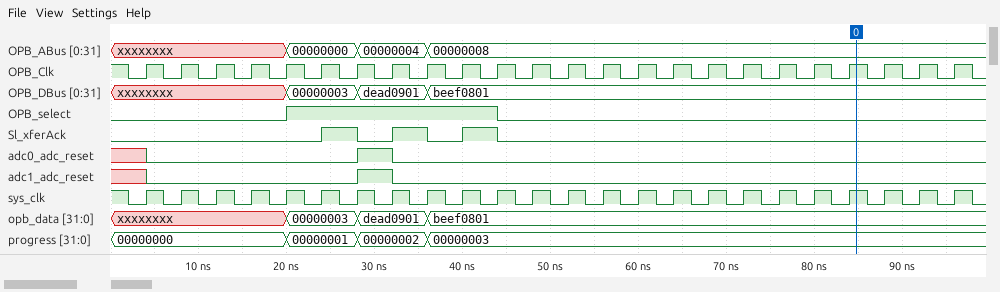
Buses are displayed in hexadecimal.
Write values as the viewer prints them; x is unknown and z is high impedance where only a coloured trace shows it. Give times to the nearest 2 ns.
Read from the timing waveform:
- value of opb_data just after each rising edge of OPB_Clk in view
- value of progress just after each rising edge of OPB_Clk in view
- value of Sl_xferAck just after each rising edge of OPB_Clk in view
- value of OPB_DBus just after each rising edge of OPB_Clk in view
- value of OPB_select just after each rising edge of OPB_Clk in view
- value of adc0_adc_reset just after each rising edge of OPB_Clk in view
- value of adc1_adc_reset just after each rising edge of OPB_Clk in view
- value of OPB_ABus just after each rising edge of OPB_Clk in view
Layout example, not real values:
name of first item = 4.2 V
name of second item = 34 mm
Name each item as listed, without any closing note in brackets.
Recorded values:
value of opb_data just after each rising edge of OPB_Clk in view = xxxxxxxx, xxxxxxxx, xxxxxxxx, xxxxxxxx, 00000003, 00000003, dead0901, dead0901, beef0801, beef0801, beef0801, beef0801, beef0801, beef0801, beef0801, beef0801, beef0801, beef0801, beef0801, beef0801, beef0801, beef0801, beef0801, beef0801
value of progress just after each rising edge of OPB_Clk in view = 00000000, 00000000, 00000000, 00000000, 00000001, 00000001, 00000002, 00000002, 00000003, 00000003, 00000003, 00000003, 00000003, 00000003, 00000003, 00000003, 00000003, 00000003, 00000003, 00000003, 00000003, 00000003, 00000003, 00000003
value of Sl_xferAck just after each rising edge of OPB_Clk in view = 0 0 0 0 0 1 0 1 0 1 0 0 0 0 0 0 0 0 0 0 0 0 0 0
value of OPB_DBus just after each rising edge of OPB_Clk in view = xxxxxxxx, xxxxxxxx, xxxxxxxx, xxxxxxxx, 00000003, 00000003, dead0901, dead0901, beef0801, beef0801, beef0801, beef0801, beef0801, beef0801, beef0801, beef0801, beef0801, beef0801, beef0801, beef0801, beef0801, beef0801, beef0801, beef0801
value of OPB_select just after each rising edge of OPB_Clk in view = 0 0 0 0 1 1 1 1 1 1 0 0 0 0 0 0 0 0 0 0 0 0 0 0
value of adc0_adc_reset just after each rising edge of OPB_Clk in view = 0 0 0 0 0 0 1 0 0 0 0 0 0 0 0 0 0 0 0 0 0 0 0 0
value of adc1_adc_reset just after each rising edge of OPB_Clk in view = 0 0 0 0 0 0 1 0 0 0 0 0 0 0 0 0 0 0 0 0 0 0 0 0
value of OPB_ABus just after each rising edge of OPB_Clk in view = xxxxxxxx, xxxxxxxx, xxxxxxxx, xxxxxxxx, 00000000, 00000000, 00000004, 00000004, 00000008, 00000008, 00000008, 00000008, 00000008, 00000008, 00000008, 00000008, 00000008, 00000008, 00000008, 00000008, 00000008, 00000008, 00000008, 00000008
